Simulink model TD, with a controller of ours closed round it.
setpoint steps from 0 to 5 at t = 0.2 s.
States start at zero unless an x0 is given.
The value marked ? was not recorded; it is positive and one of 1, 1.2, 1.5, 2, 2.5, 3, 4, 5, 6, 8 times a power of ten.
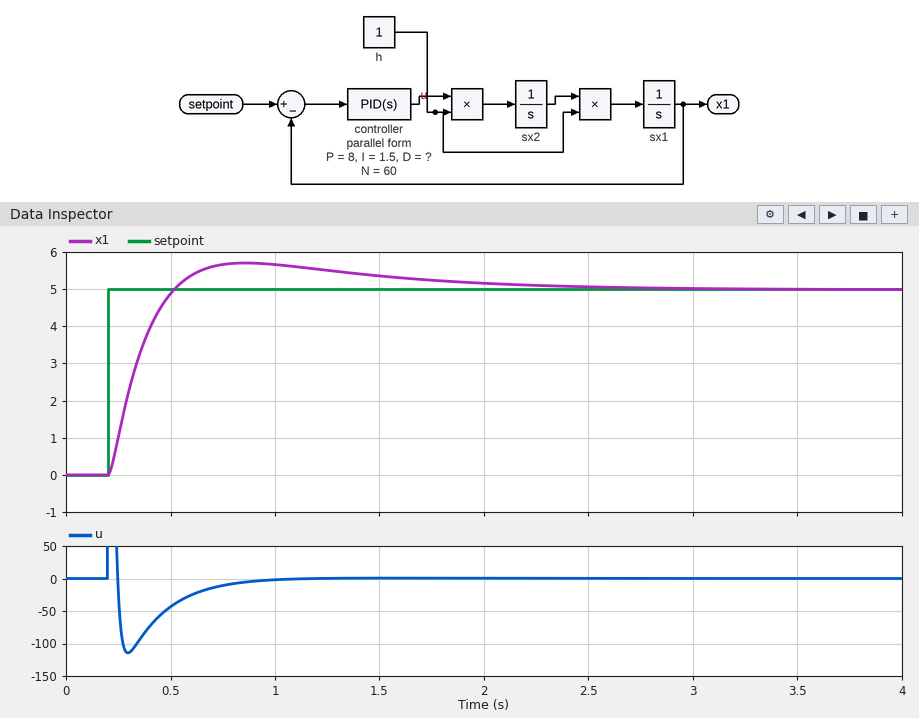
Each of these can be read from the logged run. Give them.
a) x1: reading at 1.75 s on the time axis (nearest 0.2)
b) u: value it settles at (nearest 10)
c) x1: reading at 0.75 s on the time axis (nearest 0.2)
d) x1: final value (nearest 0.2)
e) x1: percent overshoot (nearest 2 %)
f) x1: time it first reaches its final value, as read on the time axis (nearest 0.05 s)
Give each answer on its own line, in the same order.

5.2
0
5.6
5.0
14 %
0.50 s
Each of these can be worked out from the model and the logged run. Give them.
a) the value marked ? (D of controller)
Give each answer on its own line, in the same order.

6
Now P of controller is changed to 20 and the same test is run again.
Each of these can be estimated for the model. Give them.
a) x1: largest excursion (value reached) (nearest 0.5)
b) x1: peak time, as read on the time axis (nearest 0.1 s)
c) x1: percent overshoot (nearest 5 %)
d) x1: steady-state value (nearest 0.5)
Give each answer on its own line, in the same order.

6.0
0.7 s
25 %
5.0
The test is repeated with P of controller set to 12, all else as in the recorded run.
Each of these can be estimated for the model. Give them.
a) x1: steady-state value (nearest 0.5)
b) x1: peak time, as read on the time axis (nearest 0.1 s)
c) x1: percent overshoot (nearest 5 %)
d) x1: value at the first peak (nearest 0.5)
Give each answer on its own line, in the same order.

5.0
0.8 s
20 %
6.0
